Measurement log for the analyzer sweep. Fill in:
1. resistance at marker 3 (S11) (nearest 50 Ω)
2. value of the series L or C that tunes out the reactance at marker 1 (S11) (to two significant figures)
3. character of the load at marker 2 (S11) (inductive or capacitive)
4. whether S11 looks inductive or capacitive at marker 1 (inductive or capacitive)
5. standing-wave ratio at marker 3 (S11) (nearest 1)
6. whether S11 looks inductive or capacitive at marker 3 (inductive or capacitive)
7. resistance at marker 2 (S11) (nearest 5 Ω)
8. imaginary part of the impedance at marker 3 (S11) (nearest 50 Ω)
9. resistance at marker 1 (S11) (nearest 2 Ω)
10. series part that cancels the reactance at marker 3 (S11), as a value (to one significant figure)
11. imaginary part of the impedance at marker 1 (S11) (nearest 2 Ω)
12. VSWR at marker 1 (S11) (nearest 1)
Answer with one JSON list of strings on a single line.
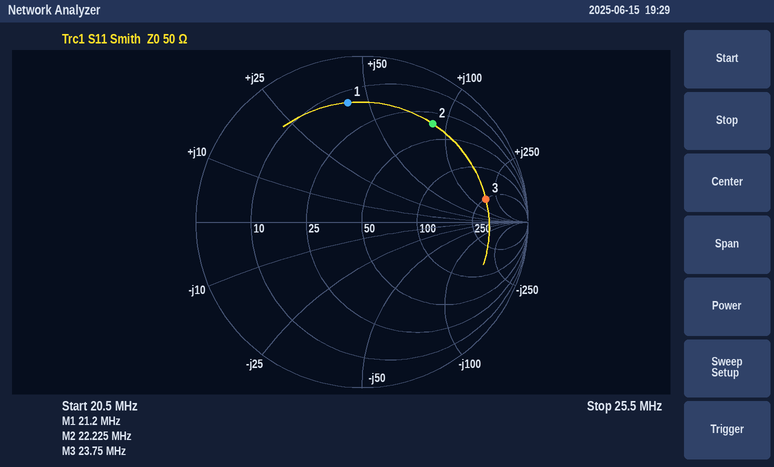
["250 Ω", "180 pF", "inductive", "inductive", "7", "inductive", "35 Ω", "+150 Ω", "14 Ω", "40 pF", "+42 Ω", "6"]
